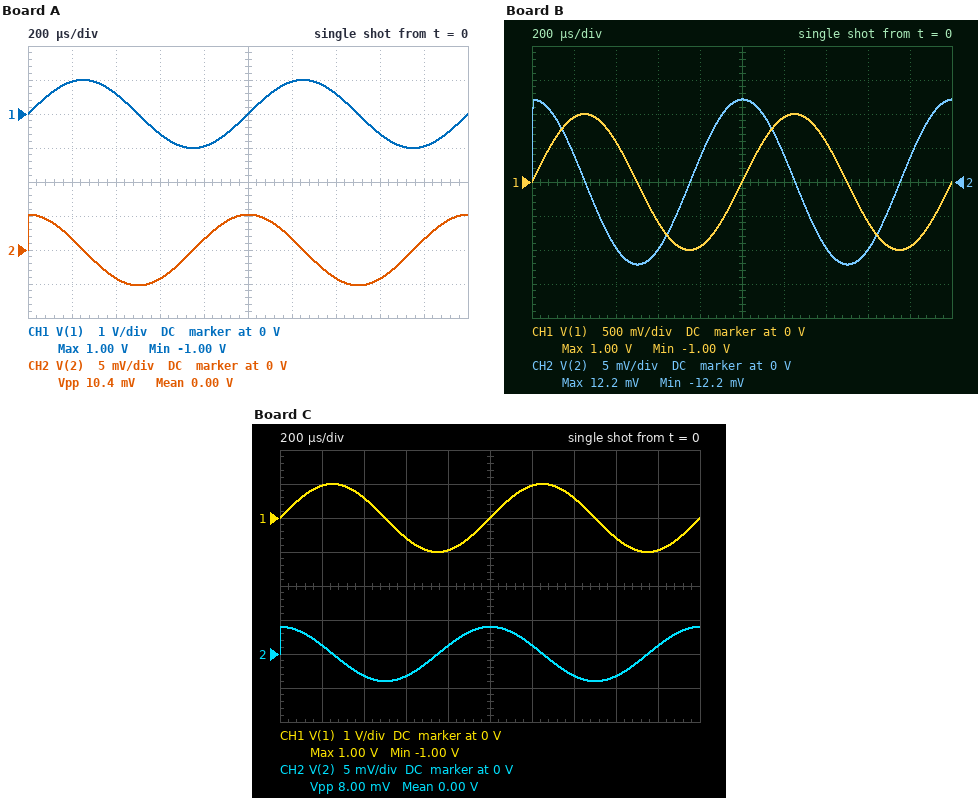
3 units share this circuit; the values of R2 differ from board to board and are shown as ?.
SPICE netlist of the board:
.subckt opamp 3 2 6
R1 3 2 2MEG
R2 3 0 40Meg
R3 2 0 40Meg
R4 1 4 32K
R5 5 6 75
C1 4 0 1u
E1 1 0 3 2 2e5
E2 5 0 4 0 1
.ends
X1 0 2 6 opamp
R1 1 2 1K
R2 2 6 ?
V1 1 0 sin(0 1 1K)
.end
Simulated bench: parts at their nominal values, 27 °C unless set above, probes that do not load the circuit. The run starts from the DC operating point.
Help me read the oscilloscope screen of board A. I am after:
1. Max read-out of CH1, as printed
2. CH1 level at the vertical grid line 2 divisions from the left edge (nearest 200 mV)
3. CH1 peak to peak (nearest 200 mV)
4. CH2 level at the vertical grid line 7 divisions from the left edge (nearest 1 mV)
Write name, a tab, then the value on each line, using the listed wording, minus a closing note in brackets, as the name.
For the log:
Max read-out of CH1, as printed	1.00 V
CH1 level at the vertical grid line 2 divisions from the left edge	600 mV
CH1 peak to peak	2.0 V
CH2 level at the vertical grid line 7 divisions from the left edge	-4 mV
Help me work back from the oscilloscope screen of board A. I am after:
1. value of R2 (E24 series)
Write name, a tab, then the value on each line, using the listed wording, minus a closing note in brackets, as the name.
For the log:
value of R2	5.1 kΩ
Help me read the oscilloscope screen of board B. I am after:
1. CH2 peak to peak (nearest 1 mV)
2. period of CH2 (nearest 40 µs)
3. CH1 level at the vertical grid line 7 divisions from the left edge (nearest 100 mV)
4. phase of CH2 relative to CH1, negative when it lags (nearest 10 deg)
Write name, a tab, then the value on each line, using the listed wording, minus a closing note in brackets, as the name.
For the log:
CH2 peak to peak	24 mV
period of CH2	1.00 ms
CH1 level at the vertical grid line 7 divisions from the left edge	600 mV
phase of CH2 relative to CH1, negative when it lags	90 deg
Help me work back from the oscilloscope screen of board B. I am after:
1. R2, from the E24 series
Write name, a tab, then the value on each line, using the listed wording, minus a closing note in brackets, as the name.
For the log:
R2, from the E24 series	12 kΩ
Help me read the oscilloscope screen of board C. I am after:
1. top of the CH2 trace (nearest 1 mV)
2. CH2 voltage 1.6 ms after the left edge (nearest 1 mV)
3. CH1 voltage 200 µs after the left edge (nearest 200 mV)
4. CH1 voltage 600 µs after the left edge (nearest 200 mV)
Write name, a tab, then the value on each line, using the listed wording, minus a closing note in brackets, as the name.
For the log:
top of the CH2 trace	4 mV
CH2 voltage 1.6 ms after the left edge	-3 mV
CH1 voltage 200 µs after the left edge	1.0 V
CH1 voltage 600 µs after the left edge	-600 mV
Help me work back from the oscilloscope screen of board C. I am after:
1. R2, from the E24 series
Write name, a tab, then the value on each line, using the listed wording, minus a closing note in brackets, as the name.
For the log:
R2, from the E24 series	3.9 kΩ
